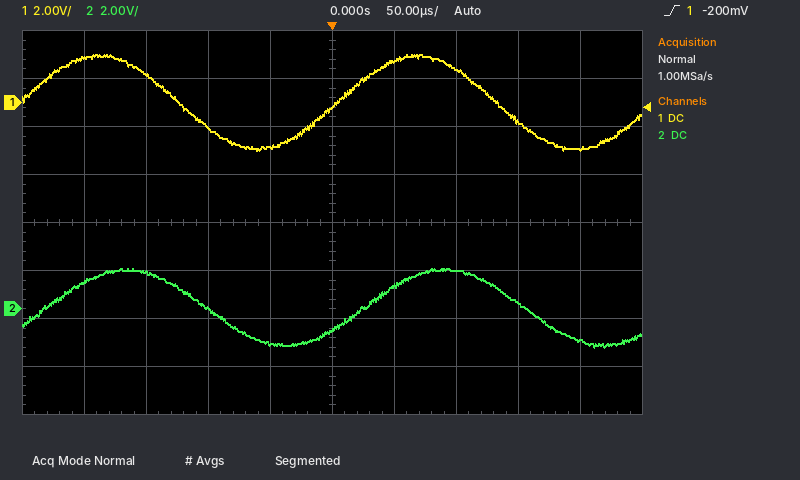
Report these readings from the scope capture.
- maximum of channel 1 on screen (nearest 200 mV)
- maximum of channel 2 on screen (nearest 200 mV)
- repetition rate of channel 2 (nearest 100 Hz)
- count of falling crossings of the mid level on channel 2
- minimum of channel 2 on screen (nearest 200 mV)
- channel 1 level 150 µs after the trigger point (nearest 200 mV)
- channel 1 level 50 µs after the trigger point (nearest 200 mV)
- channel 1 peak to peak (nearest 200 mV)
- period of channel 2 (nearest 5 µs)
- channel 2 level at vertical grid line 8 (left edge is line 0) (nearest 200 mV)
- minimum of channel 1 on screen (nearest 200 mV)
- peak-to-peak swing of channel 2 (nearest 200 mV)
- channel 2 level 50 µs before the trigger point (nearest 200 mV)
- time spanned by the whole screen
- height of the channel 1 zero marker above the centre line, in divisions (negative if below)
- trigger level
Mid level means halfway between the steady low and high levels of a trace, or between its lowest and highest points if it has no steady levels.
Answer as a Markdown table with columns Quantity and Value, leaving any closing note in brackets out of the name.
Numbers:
| Quantity | Value |
|---|---|
| maximum of channel 1 on screen | 2.0 V |
| maximum of channel 2 on screen | 1.6 V |
| repetition rate of channel 2 | 3.9 kHz |
| count of falling crossings of the mid level on channel 2 | 2 |
| minimum of channel 2 on screen | -1.6 V |
| channel 1 level 150 µs after the trigger point | -800 mV |
| channel 1 level 50 µs after the trigger point | 1.8 V |
| channel 1 peak to peak | 4.0 V |
| period of channel 2 | 255 µs |
| channel 2 level at vertical grid line 8 (left edge is line 0) | 200 mV |
| minimum of channel 1 on screen | -2.0 V |
| peak-to-peak swing of channel 2 | 3.2 V |
| channel 2 level 50 µs before the trigger point | -1.4 V |
| time spanned by the whole screen | 500 µs |
| height of the channel 1 zero marker above the centre line, in divisions | +2.5 div |
| trigger level | -200 mV |
